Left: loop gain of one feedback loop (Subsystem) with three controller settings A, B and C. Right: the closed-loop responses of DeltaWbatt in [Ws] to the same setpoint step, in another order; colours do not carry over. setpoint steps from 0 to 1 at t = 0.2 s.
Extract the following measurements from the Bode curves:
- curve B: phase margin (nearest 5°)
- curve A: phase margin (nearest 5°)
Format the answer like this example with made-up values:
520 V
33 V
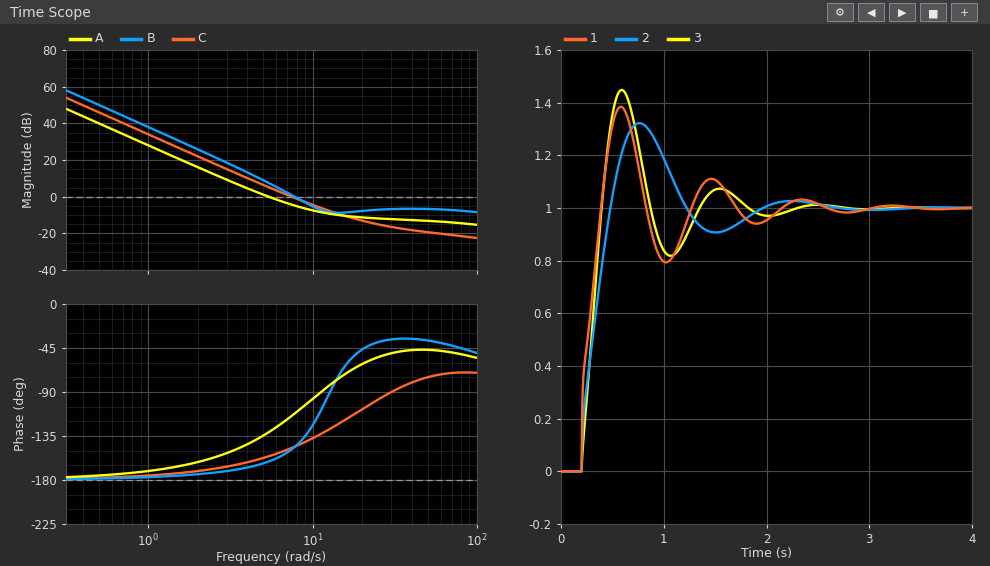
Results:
35°
50°
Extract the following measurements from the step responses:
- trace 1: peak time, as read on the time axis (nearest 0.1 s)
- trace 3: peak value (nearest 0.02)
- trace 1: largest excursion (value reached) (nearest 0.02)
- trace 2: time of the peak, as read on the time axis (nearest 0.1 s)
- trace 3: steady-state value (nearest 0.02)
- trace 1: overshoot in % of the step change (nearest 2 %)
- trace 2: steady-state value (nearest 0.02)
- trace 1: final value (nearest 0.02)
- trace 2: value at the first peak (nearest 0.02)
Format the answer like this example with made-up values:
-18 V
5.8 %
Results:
0.6 s
1.44
1.38
0.8 s
1.00
38 %
1.00
1.00
1.32
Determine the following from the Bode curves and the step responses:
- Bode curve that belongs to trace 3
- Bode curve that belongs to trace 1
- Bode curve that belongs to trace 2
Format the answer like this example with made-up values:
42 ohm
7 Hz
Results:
C
B
A
